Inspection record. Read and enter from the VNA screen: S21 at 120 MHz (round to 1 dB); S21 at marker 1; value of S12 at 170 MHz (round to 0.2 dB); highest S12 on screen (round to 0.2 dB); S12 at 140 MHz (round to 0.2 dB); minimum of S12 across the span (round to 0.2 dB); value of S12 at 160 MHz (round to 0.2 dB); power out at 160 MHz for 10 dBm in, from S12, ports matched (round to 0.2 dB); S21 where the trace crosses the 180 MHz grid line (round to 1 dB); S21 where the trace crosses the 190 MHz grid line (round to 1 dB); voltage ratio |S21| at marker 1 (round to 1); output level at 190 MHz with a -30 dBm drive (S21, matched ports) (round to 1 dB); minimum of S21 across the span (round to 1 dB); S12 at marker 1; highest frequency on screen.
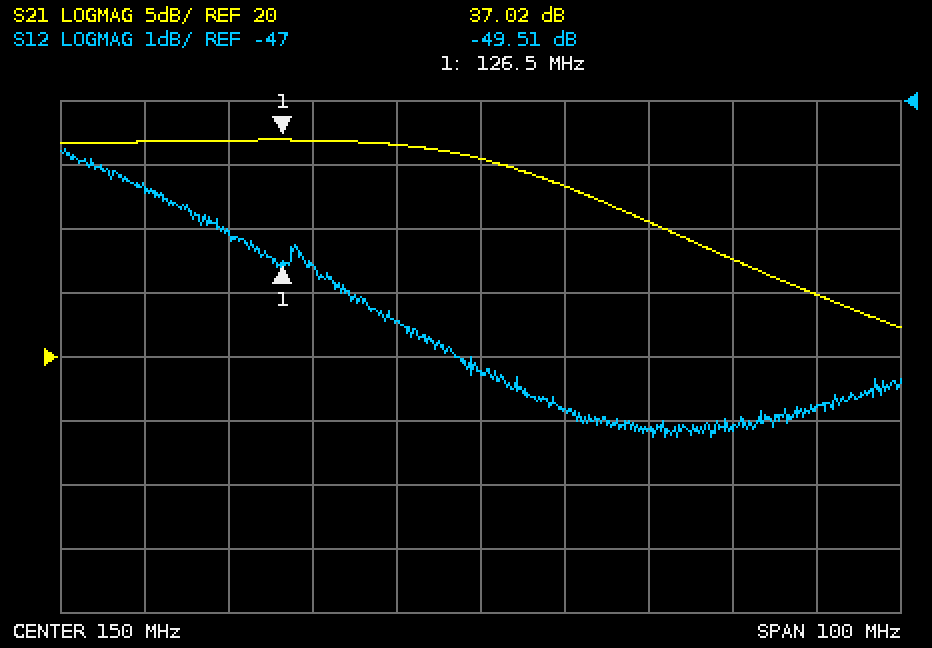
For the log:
37 dB
37.02 dB
-52.2 dB
-47.8 dB
-50.4 dB
-52.2 dB
-51.8 dB
-41.8 dBm
28 dB
25 dB
71
-5 dBm
22 dB
-49.51 dB
200 MHz
